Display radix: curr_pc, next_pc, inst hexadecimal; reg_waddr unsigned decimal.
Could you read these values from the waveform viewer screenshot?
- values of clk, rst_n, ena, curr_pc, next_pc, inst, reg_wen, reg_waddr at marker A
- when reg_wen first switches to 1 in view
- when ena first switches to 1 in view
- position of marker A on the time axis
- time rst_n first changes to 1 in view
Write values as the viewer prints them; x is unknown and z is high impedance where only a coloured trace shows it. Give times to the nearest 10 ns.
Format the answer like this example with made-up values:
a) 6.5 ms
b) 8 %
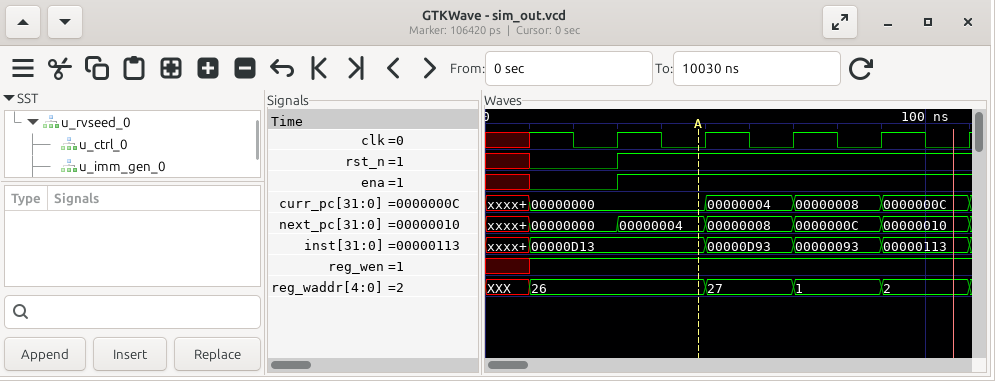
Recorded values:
a) clk=0, rst_n=1, ena=1, curr_pc=00000000, next_pc=00000004, inst=00000D13, reg_wen=1, reg_waddr=26
b) 10 ns
c) 30 ns
d) 50 ns
e) 30 ns
